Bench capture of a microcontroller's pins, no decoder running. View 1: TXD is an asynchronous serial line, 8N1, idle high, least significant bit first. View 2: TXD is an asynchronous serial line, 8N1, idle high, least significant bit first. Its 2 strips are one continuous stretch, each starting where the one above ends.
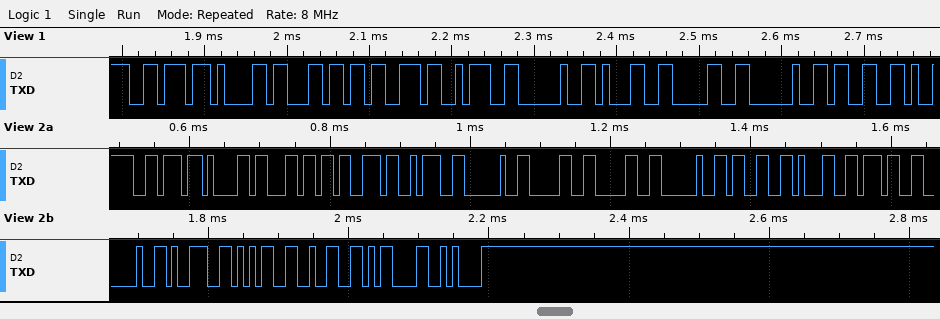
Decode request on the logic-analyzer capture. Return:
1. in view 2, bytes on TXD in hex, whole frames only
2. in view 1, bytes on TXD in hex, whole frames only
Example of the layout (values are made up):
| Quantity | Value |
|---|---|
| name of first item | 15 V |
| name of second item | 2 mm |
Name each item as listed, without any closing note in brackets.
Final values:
| Quantity | Value |
|---|---|
| in view 2, bytes on TXD in hex, whole frames only | 76 61 6C 73 3A 20 30 30 20 33 31 37 20 39 35 32 0D 0A |
| in view 1, bytes on TXD in hex, whole frames only | 0x76 0x61 0x6C 0x73 0x3A 0x20 0x31 0x30 0x20 0x33 |
